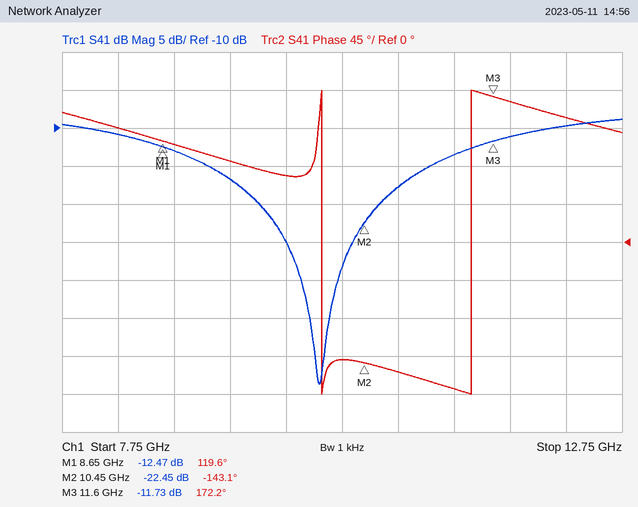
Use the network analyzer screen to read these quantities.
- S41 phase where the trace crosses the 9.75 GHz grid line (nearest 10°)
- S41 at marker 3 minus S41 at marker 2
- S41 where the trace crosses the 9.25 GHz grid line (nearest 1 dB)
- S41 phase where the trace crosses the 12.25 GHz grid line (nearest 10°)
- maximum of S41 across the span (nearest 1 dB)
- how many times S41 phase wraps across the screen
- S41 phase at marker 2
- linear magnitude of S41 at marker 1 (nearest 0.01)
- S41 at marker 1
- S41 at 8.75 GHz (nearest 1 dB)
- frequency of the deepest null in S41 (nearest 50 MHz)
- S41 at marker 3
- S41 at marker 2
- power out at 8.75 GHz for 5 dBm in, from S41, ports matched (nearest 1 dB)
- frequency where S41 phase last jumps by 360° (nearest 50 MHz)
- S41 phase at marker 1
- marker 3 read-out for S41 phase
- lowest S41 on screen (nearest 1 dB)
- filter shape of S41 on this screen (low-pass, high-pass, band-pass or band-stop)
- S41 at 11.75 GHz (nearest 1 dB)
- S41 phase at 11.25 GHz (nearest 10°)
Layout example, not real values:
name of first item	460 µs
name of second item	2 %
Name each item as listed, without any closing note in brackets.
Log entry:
S41 phase where the trace crosses the 9.75 GHz grid line	80°
S41 at marker 3 minus S41 at marker 2	10.72 dB
S41 where the trace crosses the 9.25 GHz grid line	-17 dB
S41 phase where the trace crosses the 12.25 GHz grid line	150°
maximum of S41 across the span	-9 dB
how many times S41 phase wraps across the screen	2
S41 phase at marker 2	-143.1°
linear magnitude of S41 at marker 1	0.24
S41 at marker 1	-12.47 dB
S41 at 8.75 GHz	-13 dB
frequency of the deepest null in S41	10.05 GHz
S41 at marker 3	-11.73 dB
S41 at marker 2	-22.45 dB
power out at 8.75 GHz for 5 dBm in, from S41, ports matched	-8 dBm
frequency where S41 phase last jumps by 360°	11.40 GHz
S41 phase at marker 1	119.6°
marker 3 read-out for S41 phase	172.2°
lowest S41 on screen	-44 dB
filter shape of S41 on this screen	band-stop
S41 at 11.75 GHz	-11 dB
S41 phase at 11.25 GHz	-170°
